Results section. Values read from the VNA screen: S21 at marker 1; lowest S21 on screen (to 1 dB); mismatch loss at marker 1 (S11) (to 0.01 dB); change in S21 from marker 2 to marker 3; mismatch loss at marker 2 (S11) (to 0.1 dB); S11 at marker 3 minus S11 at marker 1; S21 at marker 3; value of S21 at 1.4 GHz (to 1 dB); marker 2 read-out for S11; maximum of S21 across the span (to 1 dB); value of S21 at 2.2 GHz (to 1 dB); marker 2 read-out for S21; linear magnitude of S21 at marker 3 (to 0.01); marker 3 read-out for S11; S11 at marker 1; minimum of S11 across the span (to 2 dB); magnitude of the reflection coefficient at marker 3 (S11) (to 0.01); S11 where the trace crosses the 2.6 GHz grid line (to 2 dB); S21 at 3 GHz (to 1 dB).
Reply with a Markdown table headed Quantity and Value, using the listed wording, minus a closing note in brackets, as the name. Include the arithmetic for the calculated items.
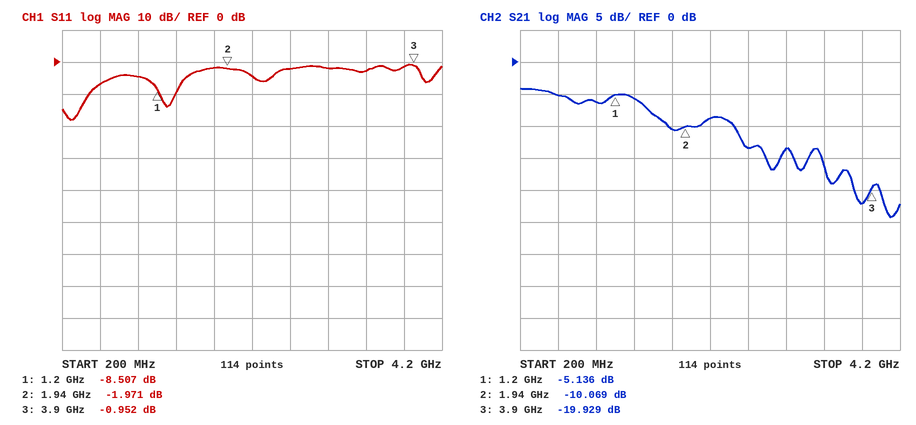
| Quantity | Value |
|---|---|
| S21 at marker 1 | -5.136 dB |
| lowest S21 on screen | -24 dB |
| mismatch loss at marker 1 (S11) | −10 log10(1 − 10^(-8.507/10)) ≈ 0.66 dB |
| change in S21 from marker 2 to marker 3 | -19.929 − (-10.069) = -9.860 dB |
| mismatch loss at marker 2 (S11) | −10 log10(1 − 10^(-1.971/10)) ≈ 4.4 dB |
| S11 at marker 3 minus S11 at marker 1 | -0.952 − (-8.507) = 7.555 dB |
| S21 at marker 3 | -19.929 dB |
| value of S21 at 1.4 GHz | -6 dB |
| marker 2 read-out for S11 | -1.971 dB |
| maximum of S21 across the span | -4 dB |
| value of S21 at 2.2 GHz | -9 dB |
| marker 2 read-out for S21 | -10.069 dB |
| linear magnitude of S21 at marker 3 | 10^(-19.929/20) ≈ 0.10 |
| marker 3 read-out for S11 | -0.952 dB |
| S11 at marker 1 | -8.507 dB |
| minimum of S11 across the span | -18 dB |
| magnitude of the reflection coefficient at marker 3 (S11) | 10^(-0.952/20) ≈ 0.90 |
| S11 where the trace crosses the 2.6 GHz grid line | -2 dB |
| S21 at 3 GHz | -14 dB |
